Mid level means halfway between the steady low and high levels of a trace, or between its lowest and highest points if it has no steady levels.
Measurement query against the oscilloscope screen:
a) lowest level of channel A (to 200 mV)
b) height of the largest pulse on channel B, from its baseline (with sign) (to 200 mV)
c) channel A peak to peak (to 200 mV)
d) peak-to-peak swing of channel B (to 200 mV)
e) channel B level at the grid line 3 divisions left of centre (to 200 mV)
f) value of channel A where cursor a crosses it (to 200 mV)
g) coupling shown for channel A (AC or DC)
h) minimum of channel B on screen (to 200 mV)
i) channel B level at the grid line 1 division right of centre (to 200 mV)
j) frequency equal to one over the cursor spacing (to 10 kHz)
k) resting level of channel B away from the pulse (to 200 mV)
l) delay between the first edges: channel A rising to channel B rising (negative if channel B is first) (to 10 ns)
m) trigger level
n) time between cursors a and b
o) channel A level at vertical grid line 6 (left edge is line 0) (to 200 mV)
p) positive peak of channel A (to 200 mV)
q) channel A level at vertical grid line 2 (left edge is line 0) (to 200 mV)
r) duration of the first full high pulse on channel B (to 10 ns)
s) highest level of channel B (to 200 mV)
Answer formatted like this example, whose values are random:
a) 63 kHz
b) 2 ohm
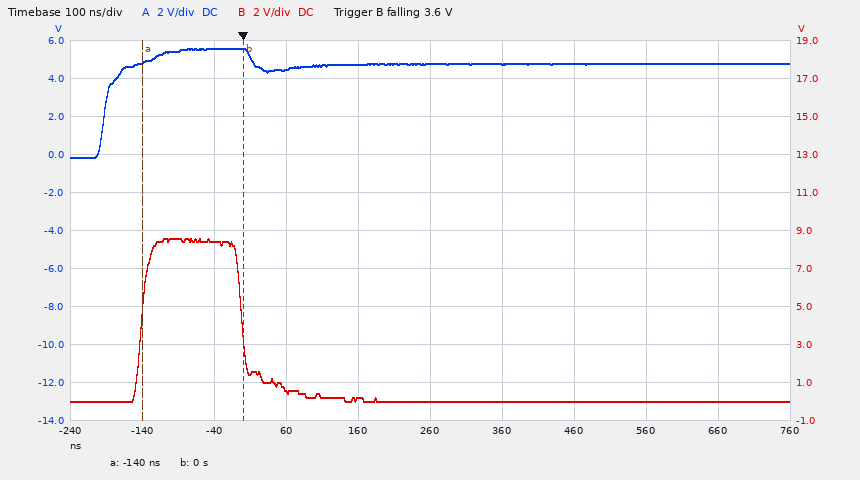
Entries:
a) -200 mV
b) +8.6 V
c) 5.8 V
d) 8.6 V
e) 8.4 V
f) 4.8 V
g) DC
h) 0.0 V
i) 0.0 V
j) 7.14 MHz
k) 0.0 V
l) +50 ns
m) 3.6 V
n) 140 ns
o) 4.8 V
p) 5.6 V
q) 5.6 V
r) 140 ns
s) 8.6 V
